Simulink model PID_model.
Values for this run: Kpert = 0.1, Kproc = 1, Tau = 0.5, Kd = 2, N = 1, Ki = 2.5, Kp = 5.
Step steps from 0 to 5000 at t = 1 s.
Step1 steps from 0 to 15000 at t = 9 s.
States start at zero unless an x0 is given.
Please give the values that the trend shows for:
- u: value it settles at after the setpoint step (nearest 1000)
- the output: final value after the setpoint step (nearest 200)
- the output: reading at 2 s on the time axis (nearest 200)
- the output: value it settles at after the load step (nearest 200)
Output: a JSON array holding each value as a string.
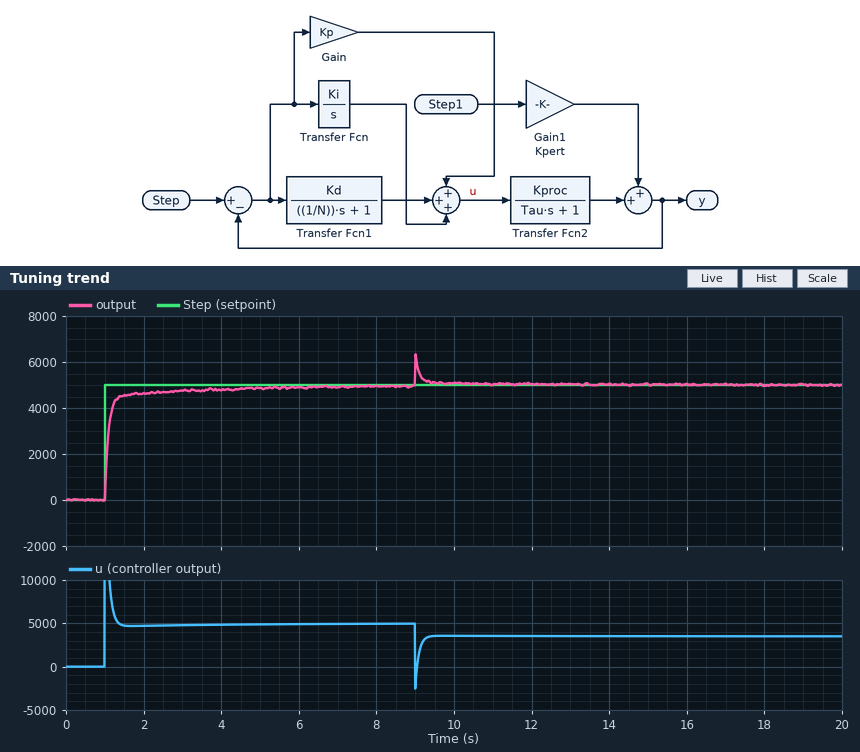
["5000", "5000", "4600", "5000"]
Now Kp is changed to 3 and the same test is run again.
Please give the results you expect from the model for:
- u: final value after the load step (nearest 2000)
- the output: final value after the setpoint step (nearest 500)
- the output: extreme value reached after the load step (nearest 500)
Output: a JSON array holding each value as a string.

["4000", "5000", "6500"]
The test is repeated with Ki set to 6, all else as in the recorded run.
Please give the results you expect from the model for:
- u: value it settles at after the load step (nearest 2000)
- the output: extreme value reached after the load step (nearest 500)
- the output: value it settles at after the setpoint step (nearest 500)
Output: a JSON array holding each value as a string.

["4000", "6500", "5000"]
